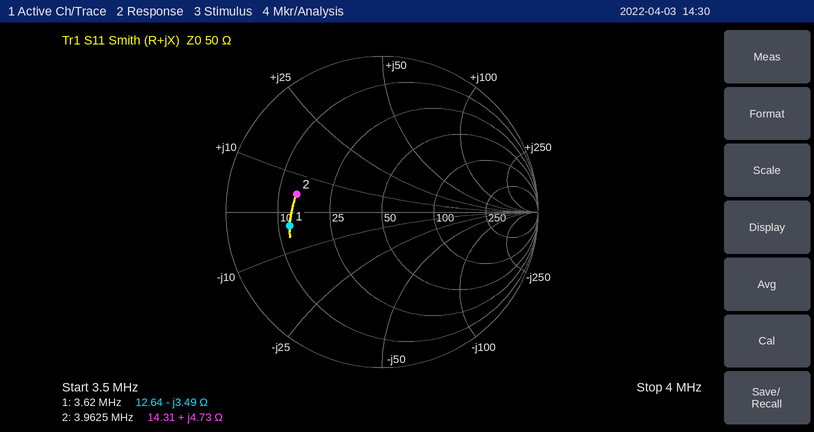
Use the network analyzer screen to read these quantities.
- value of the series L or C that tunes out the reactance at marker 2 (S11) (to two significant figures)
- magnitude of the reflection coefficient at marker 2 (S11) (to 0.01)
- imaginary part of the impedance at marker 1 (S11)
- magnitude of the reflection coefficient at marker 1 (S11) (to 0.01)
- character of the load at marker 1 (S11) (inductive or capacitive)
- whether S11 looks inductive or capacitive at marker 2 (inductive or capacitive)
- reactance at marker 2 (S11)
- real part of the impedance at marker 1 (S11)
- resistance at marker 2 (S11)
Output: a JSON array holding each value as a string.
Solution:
["8.5 nF", "0.56", "-3.49 Ω", "0.60", "capacitive", "inductive", "+4.73 Ω", "12.64 Ω", "14.31 Ω"]
